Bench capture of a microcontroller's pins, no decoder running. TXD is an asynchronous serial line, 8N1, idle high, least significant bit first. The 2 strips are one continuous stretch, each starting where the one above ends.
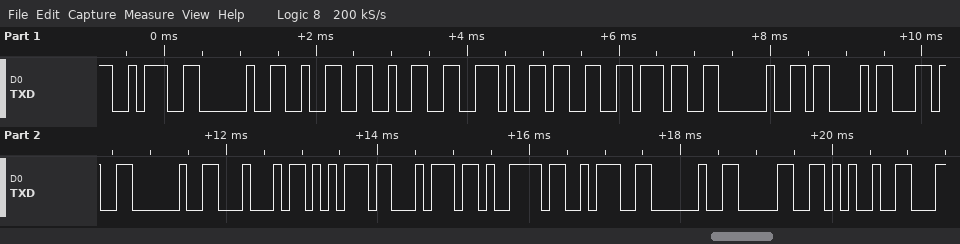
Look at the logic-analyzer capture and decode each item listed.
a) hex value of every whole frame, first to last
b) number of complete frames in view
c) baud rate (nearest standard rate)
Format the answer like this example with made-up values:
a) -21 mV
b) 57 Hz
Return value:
a) 3A 20 32 32 2E 33 37 20 43 2C 20 44 75 74 79 3A 20 30 25
b) 19
c) 9600 baud
